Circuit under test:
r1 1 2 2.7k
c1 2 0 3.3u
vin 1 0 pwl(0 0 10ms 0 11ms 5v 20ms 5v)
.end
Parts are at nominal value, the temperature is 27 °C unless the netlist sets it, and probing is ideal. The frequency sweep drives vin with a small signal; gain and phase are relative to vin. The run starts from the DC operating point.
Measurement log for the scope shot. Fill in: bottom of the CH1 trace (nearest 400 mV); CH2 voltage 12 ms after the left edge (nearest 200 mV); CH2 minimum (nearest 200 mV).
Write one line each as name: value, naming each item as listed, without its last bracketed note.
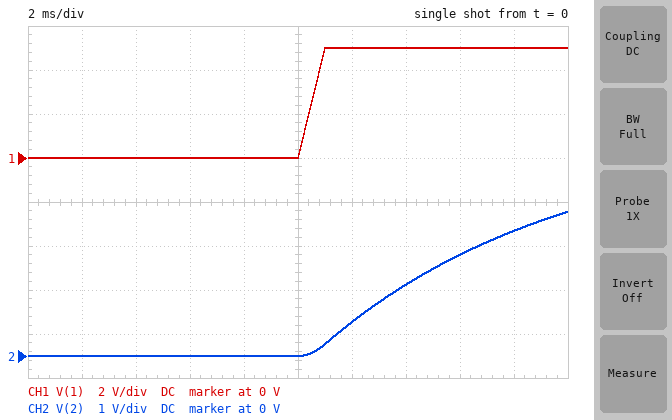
bottom of the CH1 trace: 0 V
CH2 voltage 12 ms after the left edge: 800 mV
CH2 minimum: 0 V
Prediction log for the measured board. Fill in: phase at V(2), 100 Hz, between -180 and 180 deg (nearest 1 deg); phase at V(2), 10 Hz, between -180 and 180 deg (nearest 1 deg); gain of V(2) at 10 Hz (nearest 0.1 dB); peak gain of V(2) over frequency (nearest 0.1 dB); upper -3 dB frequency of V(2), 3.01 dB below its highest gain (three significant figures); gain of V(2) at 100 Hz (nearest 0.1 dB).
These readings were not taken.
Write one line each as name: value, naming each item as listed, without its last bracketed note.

phase at V(2), 100 Hz, between -180 and 180 deg: -80 deg
phase at V(2), 10 Hz, between -180 and 180 deg: -29 deg
gain of V(2) at 10 Hz: -1.2 dB
peak gain of V(2) over frequency: 0 dB
upper -3 dB frequency of V(2), 3.01 dB below its highest gain: 17.9 Hz
gain of V(2) at 100 Hz: -15.1 dB
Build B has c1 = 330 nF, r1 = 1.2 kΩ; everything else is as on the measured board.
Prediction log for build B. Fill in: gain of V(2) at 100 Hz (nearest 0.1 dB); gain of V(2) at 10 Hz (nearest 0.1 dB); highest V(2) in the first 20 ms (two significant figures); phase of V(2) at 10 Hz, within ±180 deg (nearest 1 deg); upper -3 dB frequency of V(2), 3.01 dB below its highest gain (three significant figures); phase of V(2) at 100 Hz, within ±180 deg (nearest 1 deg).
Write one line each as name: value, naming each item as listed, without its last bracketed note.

gain of V(2) at 100 Hz: -0.3 dB
gain of V(2) at 10 Hz: 0 dB
highest V(2) in the first 20 ms: 5.0 V
phase of V(2) at 10 Hz, within ±180 deg: -1 deg
upper -3 dB frequency of V(2), 3.01 dB below its highest gain: 402 Hz
phase of V(2) at 100 Hz, within ±180 deg: -14 deg
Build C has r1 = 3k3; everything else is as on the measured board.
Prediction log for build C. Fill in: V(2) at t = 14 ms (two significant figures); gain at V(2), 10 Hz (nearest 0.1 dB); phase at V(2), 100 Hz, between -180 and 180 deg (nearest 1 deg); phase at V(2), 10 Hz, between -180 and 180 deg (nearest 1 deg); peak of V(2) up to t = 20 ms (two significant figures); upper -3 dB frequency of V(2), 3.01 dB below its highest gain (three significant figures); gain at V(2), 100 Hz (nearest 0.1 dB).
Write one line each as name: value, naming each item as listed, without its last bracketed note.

V(2) at t = 14 ms: 1.4 V
gain at V(2), 10 Hz: -1.7 dB
phase at V(2), 100 Hz, between -180 and 180 deg: -82 deg
phase at V(2), 10 Hz, between -180 and 180 deg: -34 deg
peak of V(2) up to t = 20 ms: 2.9 V
upper -3 dB frequency of V(2), 3.01 dB below its highest gain: 14.6 Hz
gain at V(2), 100 Hz: -16.8 dB
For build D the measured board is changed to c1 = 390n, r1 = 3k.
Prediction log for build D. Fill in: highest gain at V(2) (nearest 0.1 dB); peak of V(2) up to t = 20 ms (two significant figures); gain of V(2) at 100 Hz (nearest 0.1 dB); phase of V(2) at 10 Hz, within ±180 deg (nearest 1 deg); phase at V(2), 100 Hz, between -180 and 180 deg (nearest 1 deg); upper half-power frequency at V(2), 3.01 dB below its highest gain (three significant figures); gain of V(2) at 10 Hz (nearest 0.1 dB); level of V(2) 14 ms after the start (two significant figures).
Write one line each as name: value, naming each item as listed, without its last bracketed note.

highest gain at V(2): 0 dB
peak of V(2) up to t = 20 ms: 5.0 V
gain of V(2) at 100 Hz: -1.9 dB
phase of V(2) at 10 Hz, within ±180 deg: -4 deg
phase at V(2), 100 Hz, between -180 and 180 deg: -36 deg
upper half-power frequency at V(2), 3.01 dB below its highest gain: 136 Hz
gain of V(2) at 10 Hz: 0 dB
level of V(2) 14 ms after the start: 4.7 V
